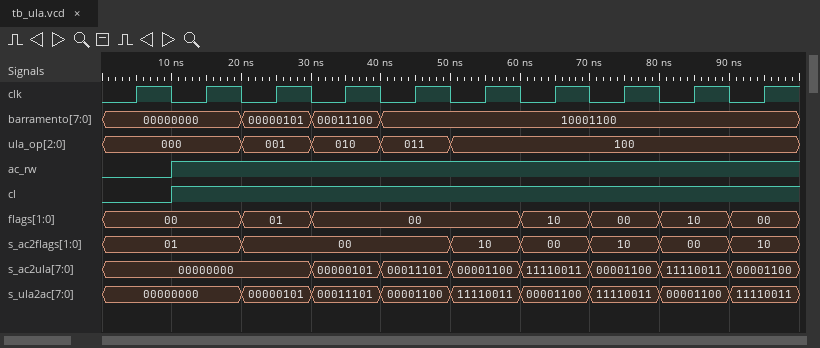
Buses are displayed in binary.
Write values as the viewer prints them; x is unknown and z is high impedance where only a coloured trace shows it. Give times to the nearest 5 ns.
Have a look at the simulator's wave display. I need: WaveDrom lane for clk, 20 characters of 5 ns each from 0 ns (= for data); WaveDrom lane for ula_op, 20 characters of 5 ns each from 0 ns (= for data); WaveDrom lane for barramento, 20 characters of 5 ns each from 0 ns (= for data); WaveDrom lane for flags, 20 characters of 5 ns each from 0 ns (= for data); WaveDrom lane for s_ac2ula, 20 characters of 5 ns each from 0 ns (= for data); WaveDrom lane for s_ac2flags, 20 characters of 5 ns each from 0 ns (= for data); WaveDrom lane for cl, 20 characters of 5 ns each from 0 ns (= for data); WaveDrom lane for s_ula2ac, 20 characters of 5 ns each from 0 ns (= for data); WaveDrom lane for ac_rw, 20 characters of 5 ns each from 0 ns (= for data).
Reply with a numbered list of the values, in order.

1. {name: 'clk', wave: '01010101010101010101'}
2. {name: 'ula_op', wave: '=...=.=.=.=.........', data: '000 001 010 011 100'}
3. {name: 'barramento', wave: '=...=.=.=...........', data: '00000000 00000101 00011100 10001100'}
4. {name: 'flags', wave: '=...=.=.....=.=.=.=.', data: '00 01 00 10 00 10 00'}
5. {name: 's_ac2ula', wave: '=.....=.=.=.=.=.=.=.', data: '00000000 00000101 00011101 00001100 11110011 00001100 11110011 00001100'}
6. {name: 's_ac2flags', wave: '=...=.....=.=.=.=.=.', data: '01 00 10 00 10 00 10'}
7. {name: 'cl', wave: '0.1.................'}
8. {name: 's_ula2ac', wave: '=...=.=.=.=.=.=.=.=.', data: '00000000 00000101 00011101 00001100 11110011 00001100 11110011 00001100 11110011'}
9. {name: 'ac_rw', wave: '0.1.................'}
